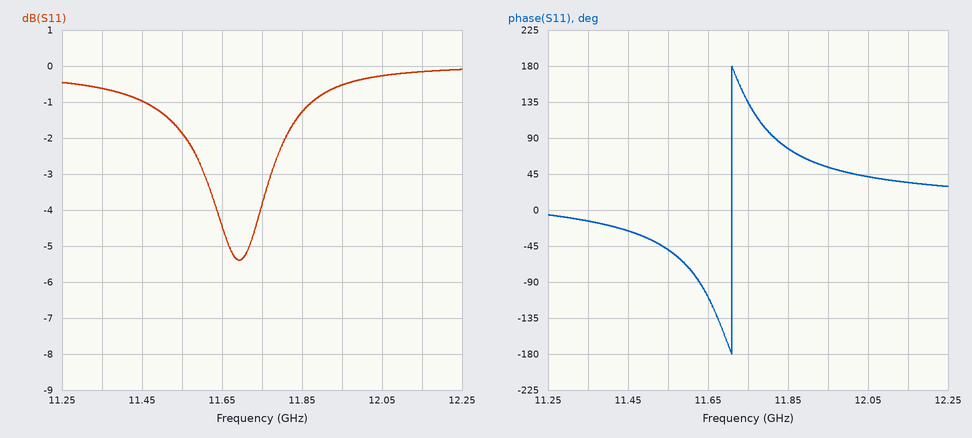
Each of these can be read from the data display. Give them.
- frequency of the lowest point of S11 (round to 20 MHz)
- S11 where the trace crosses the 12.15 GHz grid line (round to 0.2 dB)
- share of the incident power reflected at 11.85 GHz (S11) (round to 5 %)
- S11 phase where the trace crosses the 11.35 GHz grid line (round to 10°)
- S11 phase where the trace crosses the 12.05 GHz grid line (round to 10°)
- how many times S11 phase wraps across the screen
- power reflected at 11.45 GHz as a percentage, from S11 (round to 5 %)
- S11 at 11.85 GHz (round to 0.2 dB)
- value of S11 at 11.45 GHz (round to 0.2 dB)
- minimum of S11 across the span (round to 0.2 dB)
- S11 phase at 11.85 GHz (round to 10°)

11.70 GHz
-0.2 dB
75 %
-10°
40°
1
80 %
-1.2 dB
-1.0 dB
-5.4 dB
80°
